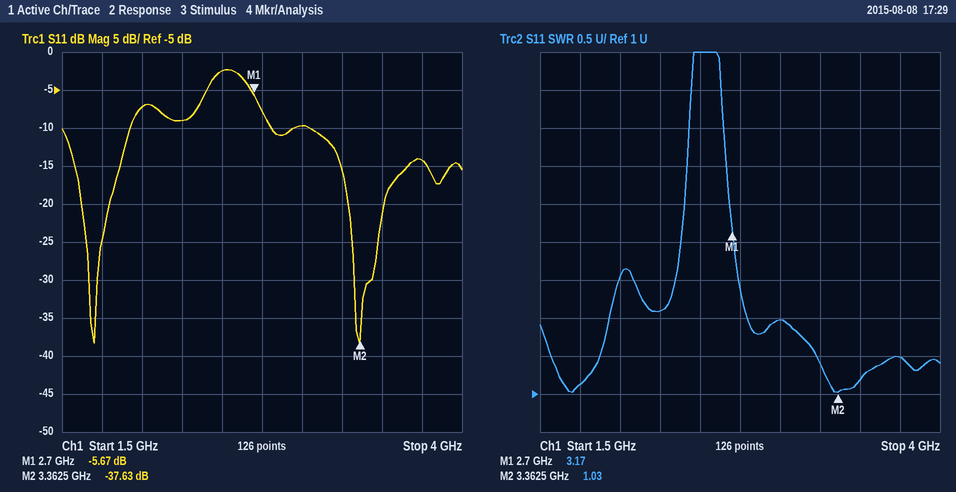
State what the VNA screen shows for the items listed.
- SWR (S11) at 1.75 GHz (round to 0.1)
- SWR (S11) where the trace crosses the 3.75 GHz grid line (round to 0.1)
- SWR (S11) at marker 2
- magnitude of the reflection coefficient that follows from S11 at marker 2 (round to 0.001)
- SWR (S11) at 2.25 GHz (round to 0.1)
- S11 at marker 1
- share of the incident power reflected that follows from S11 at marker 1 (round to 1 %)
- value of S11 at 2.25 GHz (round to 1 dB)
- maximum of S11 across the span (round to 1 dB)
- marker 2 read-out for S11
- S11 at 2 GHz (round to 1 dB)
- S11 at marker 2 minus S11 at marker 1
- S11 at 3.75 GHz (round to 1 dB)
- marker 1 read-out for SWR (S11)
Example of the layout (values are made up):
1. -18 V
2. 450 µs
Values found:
1. 1.1
2. 1.5
3. 1.03
4. 0.013
5. 2.1
6. -5.67 dB
7. 27 %
8. -9 dB
9. -2 dB
10. -37.63 dB
11. -7 dB
12. -31.96 dB
13. -14 dB
14. 3.17
